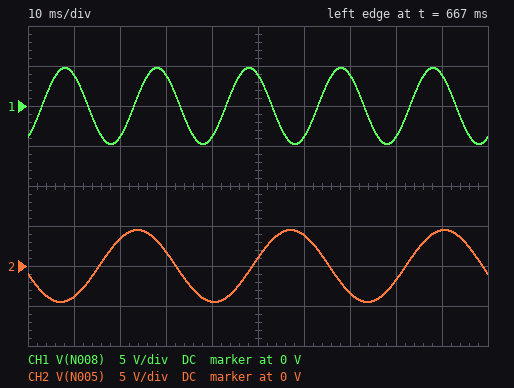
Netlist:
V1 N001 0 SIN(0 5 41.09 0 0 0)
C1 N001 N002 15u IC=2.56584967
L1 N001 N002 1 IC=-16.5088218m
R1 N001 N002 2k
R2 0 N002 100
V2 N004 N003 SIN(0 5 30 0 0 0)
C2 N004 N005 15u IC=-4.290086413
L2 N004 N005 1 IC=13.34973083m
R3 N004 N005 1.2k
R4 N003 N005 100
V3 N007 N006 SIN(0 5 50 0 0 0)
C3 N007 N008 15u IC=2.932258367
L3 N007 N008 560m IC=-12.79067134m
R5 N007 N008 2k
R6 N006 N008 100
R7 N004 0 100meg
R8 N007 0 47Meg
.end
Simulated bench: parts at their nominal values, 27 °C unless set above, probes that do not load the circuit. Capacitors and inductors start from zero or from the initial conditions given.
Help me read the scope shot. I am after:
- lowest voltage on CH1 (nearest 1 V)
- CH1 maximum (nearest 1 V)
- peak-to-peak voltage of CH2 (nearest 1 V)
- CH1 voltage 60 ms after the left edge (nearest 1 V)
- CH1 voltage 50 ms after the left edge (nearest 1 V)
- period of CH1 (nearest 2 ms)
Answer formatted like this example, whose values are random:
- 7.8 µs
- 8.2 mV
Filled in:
- -5 V
- 5 V
- 9 V
- -4 V
- 4 V
- 20 ms
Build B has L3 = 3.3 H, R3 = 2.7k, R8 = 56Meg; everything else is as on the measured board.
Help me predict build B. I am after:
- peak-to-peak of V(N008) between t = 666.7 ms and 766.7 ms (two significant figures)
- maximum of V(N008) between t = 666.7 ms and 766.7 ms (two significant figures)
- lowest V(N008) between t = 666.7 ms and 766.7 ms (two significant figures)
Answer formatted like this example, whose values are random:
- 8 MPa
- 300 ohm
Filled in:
- 9.0 V
- 4.5 V
- -4.5 V
